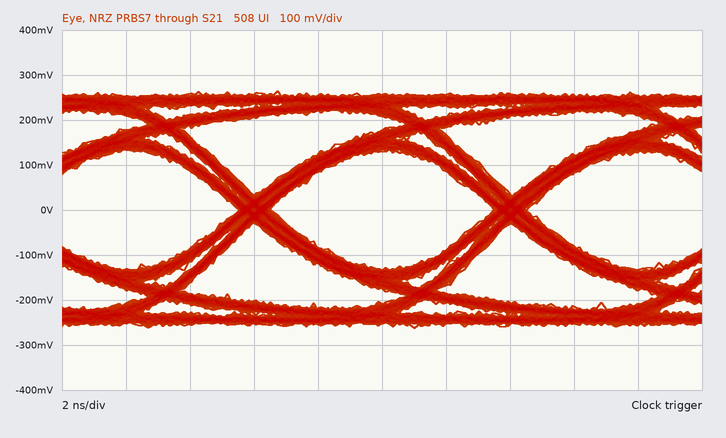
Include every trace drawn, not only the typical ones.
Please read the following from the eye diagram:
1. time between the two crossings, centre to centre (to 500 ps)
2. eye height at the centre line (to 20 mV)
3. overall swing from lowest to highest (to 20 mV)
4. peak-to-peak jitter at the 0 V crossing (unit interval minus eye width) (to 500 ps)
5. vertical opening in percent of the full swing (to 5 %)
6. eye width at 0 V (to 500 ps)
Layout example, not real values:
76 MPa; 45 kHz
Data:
8.0 ns; 260 mV; 520 mV; 1.0 ns; 50 %; 7.0 ns
